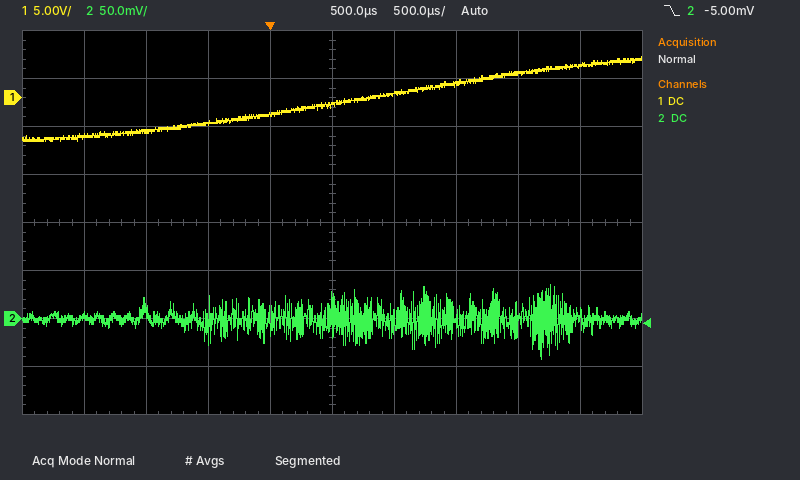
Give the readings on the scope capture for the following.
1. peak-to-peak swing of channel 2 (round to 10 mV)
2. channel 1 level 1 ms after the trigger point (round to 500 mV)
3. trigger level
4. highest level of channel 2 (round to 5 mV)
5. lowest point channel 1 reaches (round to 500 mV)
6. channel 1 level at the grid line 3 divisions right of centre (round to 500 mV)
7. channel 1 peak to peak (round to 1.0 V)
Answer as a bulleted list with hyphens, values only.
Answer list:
- 80 mV
- 500 mV
- -5.00 mV
- 35 mV
- -4.5 V
- 2.5 V
- 9.0 V
